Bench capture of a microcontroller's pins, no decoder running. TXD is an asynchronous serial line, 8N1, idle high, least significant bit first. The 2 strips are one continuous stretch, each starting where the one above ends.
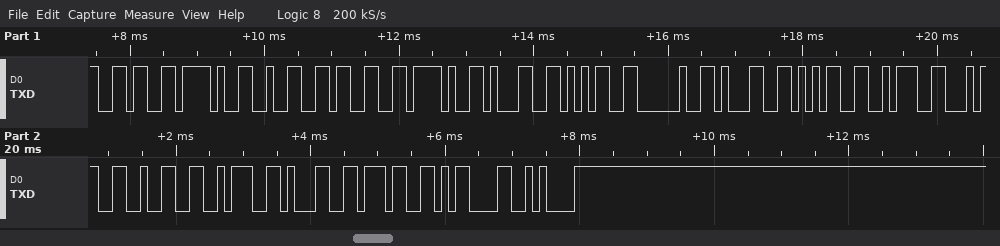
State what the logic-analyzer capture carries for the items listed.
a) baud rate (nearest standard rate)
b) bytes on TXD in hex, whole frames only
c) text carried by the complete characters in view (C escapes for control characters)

9600 baud
36 2F 32 33 2F 31 35 20 31 35 3A 34 32 3A 31 37 0D 0A
"6/23/15 15:42:17\r\n"
